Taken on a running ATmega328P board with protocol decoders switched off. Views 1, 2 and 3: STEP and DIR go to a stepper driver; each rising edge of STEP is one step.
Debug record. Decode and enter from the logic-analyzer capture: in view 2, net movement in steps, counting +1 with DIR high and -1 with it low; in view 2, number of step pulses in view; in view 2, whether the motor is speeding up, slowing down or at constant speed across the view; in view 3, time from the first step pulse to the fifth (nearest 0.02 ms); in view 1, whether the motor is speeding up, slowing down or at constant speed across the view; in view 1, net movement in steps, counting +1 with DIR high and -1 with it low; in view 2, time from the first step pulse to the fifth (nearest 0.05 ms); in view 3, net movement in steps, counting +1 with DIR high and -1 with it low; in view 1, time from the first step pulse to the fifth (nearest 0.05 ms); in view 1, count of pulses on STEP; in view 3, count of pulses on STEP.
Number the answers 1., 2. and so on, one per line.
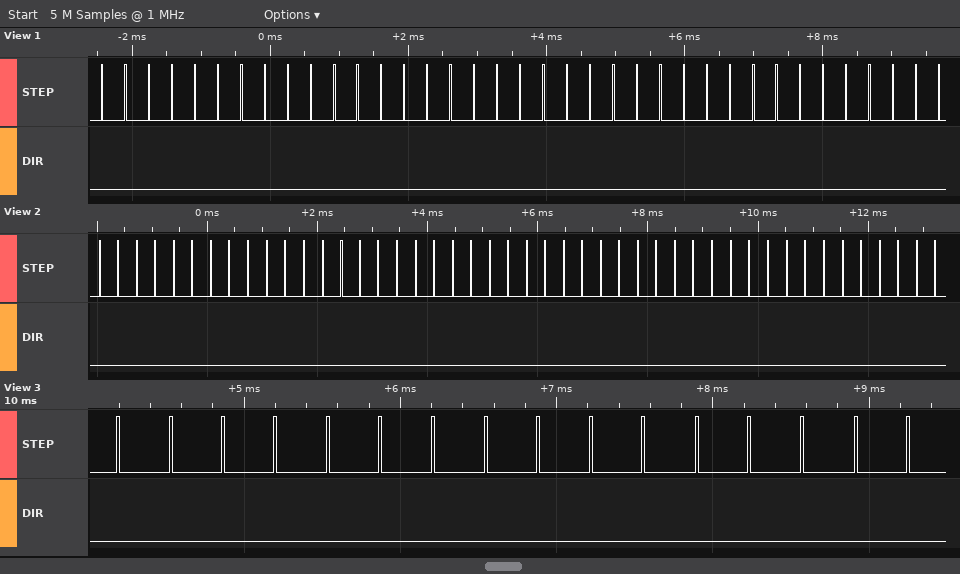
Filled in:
1. -46
2. 46
3. constant speed
4. 1.34 ms
5. constant speed
6. -37
7. 1.35 ms
8. -16
9. 1.35 ms
10. 37
11. 16
